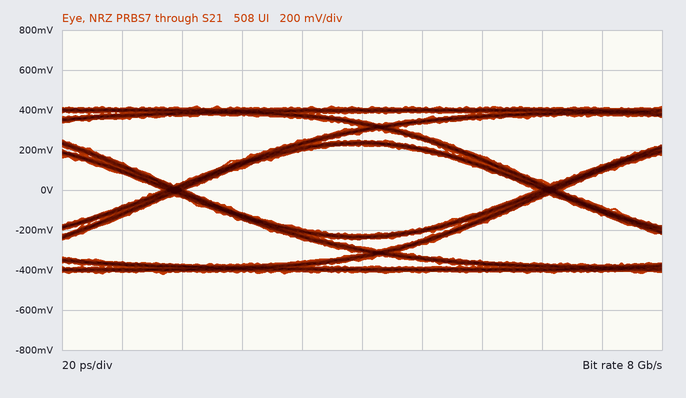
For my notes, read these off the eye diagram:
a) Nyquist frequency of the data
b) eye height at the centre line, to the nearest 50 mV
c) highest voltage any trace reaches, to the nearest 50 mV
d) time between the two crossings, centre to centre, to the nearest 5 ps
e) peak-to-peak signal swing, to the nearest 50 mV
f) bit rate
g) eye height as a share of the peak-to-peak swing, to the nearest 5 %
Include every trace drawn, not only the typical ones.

4 GHz
450 mV
400 mV
125 ps
850 mV
8 Gb/s
55 %
